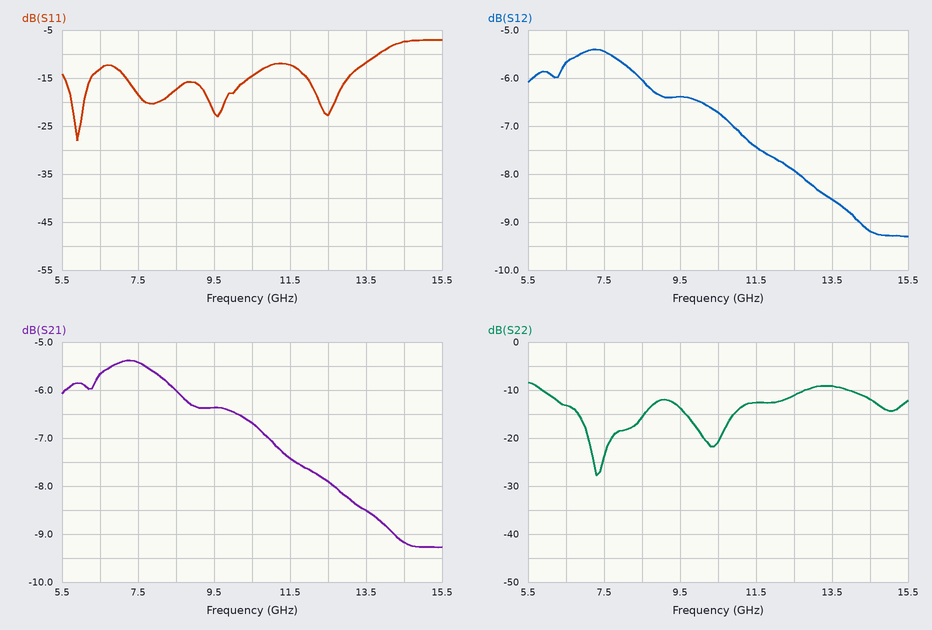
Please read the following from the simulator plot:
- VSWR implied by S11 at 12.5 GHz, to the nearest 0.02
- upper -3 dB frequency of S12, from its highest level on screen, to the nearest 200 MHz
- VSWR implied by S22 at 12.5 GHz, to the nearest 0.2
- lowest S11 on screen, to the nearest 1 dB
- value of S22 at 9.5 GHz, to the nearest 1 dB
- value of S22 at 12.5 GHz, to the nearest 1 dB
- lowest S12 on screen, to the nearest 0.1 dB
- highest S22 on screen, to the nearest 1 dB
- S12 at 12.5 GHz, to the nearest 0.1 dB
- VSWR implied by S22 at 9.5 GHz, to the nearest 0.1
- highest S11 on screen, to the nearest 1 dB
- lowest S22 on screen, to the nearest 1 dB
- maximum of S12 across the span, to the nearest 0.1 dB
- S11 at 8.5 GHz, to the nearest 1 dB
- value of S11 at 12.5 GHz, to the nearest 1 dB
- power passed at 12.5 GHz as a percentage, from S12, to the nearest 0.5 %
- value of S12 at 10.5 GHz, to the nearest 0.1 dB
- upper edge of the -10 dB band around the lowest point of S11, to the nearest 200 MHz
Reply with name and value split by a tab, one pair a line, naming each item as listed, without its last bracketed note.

VSWR implied by S11 at 12.5 GHz, to the nearest 0.02	1.16
upper -3 dB frequency of S12, from its highest level on screen, to the nearest 200 MHz	13.2 GHz
VSWR implied by S22 at 12.5 GHz, to the nearest 0.2	1.8
lowest S11 on screen, to the nearest 1 dB	-28 dB
value of S22 at 9.5 GHz, to the nearest 1 dB	-14 dB
value of S22 at 12.5 GHz, to the nearest 1 dB	-11 dB
lowest S12 on screen, to the nearest 0.1 dB	-9.3 dB
highest S22 on screen, to the nearest 1 dB	-8 dB
S12 at 12.5 GHz, to the nearest 0.1 dB	-7.9 dB
VSWR implied by S22 at 9.5 GHz, to the nearest 0.1	1.5
highest S11 on screen, to the nearest 1 dB	-7 dB
lowest S22 on screen, to the nearest 1 dB	-28 dB
maximum of S12 across the span, to the nearest 0.1 dB	-5.4 dB
S11 at 8.5 GHz, to the nearest 1 dB	-17 dB
value of S11 at 12.5 GHz, to the nearest 1 dB	-23 dB
power passed at 12.5 GHz as a percentage, from S12, to the nearest 0.5 %	16.0 %
value of S12 at 10.5 GHz, to the nearest 0.1 dB	-6.7 dB
upper edge of the -10 dB band around the lowest point of S11, to the nearest 200 MHz	13.8 GHz
